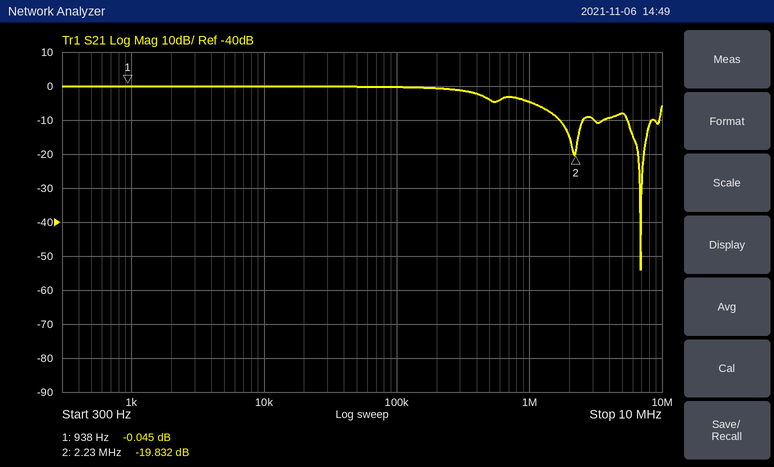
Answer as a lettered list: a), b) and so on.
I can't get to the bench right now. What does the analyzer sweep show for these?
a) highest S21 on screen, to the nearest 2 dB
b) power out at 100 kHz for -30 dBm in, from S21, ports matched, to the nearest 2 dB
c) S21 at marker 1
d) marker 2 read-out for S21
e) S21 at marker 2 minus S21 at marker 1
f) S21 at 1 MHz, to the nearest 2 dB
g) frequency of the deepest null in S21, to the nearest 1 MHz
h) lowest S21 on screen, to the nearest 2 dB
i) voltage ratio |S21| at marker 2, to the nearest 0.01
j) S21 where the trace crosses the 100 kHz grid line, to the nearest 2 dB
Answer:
a) 0 dB
b) -30 dBm
c) -0.045 dB
d) -19.832 dB
e) -19.787 dB
f) -4 dB
g) 7 MHz
h) -54 dB
i) 0.10
j) 0 dB
